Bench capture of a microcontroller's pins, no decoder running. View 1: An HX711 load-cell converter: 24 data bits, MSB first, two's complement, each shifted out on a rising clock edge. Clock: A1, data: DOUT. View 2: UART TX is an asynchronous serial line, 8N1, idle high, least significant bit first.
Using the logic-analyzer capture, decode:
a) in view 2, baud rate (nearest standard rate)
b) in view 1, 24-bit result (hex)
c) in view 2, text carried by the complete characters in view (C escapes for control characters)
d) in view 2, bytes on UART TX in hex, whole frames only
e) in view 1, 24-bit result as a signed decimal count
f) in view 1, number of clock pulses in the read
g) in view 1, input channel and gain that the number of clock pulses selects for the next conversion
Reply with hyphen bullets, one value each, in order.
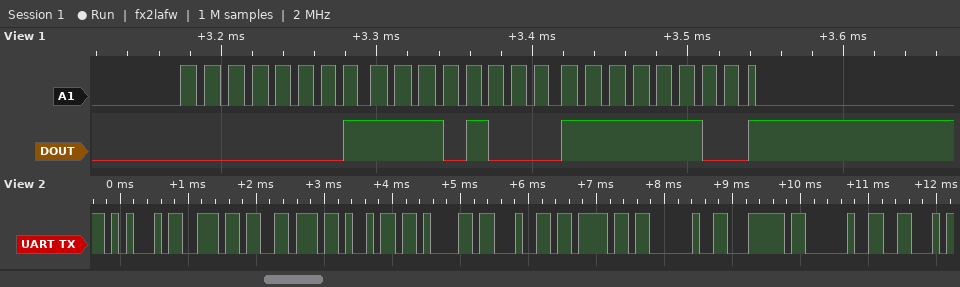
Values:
- 9600 baud
- 0x01E8FC
- "Enviado | F"
- 45 6E 76 69 61 64 6F 20 7C 20 46
- 125180
- 25
- channel A, gain 128
